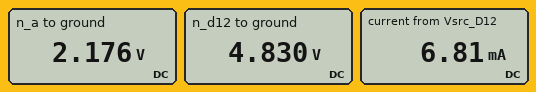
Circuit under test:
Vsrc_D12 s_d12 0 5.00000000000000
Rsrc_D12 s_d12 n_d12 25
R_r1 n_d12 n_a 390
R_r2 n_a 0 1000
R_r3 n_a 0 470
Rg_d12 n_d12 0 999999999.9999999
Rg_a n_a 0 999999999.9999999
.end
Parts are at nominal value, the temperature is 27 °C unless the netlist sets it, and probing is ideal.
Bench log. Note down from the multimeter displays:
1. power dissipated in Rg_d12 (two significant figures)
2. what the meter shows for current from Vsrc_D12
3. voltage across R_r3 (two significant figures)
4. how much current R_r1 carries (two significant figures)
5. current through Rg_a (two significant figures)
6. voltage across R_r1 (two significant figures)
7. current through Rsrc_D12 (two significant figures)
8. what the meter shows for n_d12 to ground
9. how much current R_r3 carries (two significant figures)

23 nW
6.81 mA
2.2 V
6.8 mA
2.2 nA
2.7 V
6.8 mA
4.830 V
4.6 mA
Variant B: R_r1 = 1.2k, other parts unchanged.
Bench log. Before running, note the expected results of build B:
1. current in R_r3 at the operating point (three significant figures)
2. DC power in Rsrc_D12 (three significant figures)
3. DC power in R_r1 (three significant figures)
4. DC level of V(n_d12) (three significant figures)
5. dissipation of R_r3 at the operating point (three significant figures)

2.20 mA
262 µW
12.6 mW
4.92 V
2.28 mW
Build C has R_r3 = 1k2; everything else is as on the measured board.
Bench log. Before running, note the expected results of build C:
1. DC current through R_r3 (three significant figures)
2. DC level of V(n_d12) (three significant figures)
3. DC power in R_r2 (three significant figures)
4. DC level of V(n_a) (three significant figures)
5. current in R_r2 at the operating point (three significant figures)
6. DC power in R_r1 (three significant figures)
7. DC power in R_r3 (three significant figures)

2.37 mA
4.87 V
8.06 mW
2.84 V
2.84 mA
10.6 mW
6.72 mW
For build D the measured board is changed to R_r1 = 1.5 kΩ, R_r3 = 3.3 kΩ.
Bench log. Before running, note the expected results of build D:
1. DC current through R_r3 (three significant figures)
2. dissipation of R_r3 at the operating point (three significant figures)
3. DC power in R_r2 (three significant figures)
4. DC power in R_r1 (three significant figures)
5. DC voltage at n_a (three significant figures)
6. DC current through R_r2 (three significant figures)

507 µA
849 µW
2.80 mW
7.14 mW
1.67 V
1.67 mA
